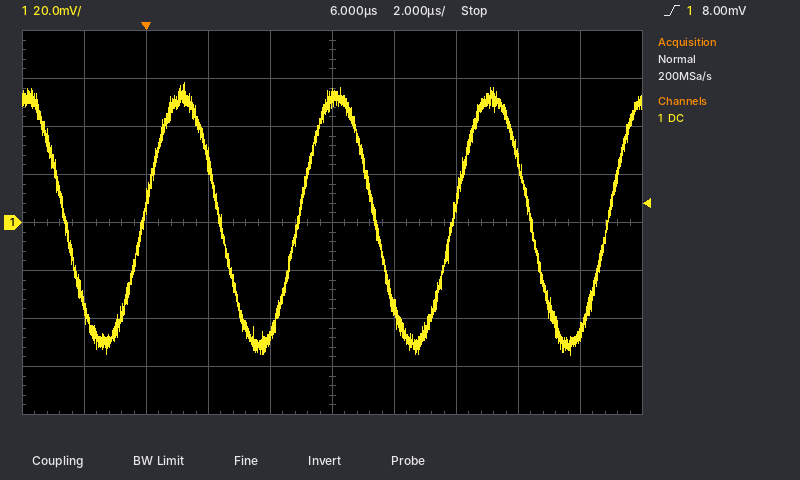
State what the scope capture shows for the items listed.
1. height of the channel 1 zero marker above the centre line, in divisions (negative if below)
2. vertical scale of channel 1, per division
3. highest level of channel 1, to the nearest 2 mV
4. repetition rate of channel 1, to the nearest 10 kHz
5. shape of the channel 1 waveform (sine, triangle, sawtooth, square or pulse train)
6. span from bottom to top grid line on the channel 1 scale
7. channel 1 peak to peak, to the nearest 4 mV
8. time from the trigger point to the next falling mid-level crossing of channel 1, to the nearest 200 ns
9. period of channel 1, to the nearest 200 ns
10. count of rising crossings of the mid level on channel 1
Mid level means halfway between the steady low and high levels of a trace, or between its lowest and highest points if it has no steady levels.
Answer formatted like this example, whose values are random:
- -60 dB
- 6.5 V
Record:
- 0.0 div
- 20 mV
- 58 mV
- 200 kHz
- sine
- 160 mV
- 112 mV
- 2.4 µs
- 5.0 µs
- 4
